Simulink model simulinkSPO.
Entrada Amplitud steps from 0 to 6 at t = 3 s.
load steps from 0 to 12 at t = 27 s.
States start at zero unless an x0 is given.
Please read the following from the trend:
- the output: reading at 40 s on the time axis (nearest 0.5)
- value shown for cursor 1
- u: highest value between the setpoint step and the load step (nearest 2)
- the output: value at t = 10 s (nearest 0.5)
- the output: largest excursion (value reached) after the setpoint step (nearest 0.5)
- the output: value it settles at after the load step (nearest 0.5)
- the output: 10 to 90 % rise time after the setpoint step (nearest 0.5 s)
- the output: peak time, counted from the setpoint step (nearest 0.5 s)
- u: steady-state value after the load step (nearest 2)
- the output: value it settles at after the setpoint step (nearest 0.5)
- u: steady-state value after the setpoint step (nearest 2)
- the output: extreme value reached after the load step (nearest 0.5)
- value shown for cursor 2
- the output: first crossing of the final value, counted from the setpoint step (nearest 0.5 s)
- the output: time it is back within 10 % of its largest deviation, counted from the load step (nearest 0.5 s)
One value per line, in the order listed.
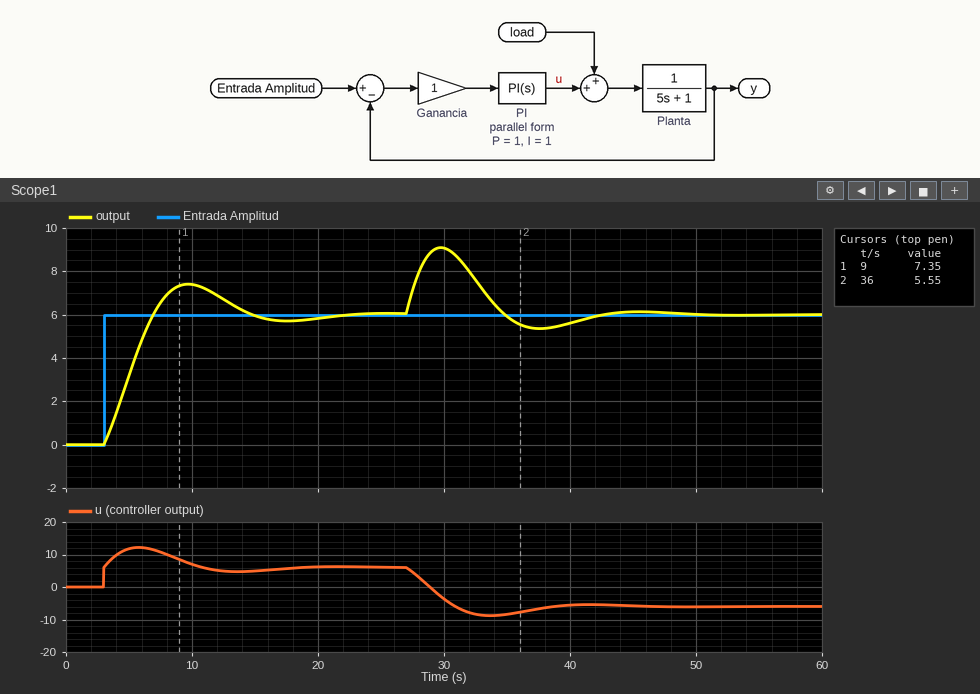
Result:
5.5
7.35
12
7.5
7.5
6.0
3.0 s
6.5 s
-6
6.0
6
9.0
5.55
4.0 s
13.5 s
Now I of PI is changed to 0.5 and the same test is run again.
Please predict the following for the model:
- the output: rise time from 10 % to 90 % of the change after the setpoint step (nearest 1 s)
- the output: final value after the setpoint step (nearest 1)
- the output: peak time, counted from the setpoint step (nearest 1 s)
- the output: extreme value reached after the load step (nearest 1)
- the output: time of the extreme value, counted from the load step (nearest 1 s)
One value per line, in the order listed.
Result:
5 s
6
10 s
10
4 s
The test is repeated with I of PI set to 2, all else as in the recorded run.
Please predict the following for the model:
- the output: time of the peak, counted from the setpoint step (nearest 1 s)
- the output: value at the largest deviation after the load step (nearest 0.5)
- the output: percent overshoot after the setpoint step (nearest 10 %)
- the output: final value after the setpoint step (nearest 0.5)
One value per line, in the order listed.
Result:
5 s
8.5
40 %
6.0
